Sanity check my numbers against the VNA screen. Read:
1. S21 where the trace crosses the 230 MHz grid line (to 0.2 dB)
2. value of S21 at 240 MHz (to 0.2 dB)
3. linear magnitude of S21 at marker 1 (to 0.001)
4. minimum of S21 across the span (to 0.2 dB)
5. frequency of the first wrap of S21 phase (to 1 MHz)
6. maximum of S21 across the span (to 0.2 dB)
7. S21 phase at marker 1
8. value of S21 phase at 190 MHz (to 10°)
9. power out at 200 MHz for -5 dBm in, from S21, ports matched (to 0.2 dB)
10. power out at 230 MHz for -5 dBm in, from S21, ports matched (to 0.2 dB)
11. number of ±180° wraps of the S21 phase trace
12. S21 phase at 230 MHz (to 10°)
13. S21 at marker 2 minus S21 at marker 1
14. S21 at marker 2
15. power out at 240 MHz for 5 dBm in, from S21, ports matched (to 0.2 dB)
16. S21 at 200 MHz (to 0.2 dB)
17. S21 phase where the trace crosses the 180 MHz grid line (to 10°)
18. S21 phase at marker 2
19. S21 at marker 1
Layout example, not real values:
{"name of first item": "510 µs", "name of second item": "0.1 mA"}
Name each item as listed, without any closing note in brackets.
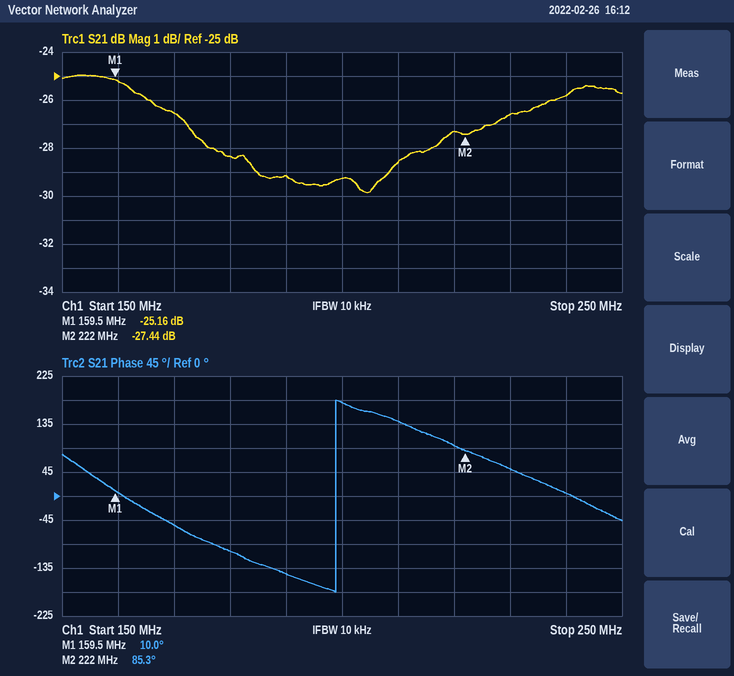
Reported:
{"S21 where the trace crosses the 230 MHz grid line": "-26.6 dB", "value of S21 at 240 MHz": "-25.8 dB", "linear magnitude of S21 at marker 1": "0.055", "minimum of S21 across the span": "-29.8 dB", "frequency of the first wrap of S21 phase": "199 MHz", "maximum of S21 across the span": "-25.0 dB", "S21 phase at marker 1": "10.0°", "value of S21 phase at 190 MHz": "-150°", "power out at 200 MHz for -5 dBm in, from S21, ports matched": "-34.2 dBm", "power out at 230 MHz for -5 dBm in, from S21, ports matched": "-31.6 dBm", "number of ±180° wraps of the S21 phase trace": "1", "S21 phase at 230 MHz": "50°", "S21 at marker 2 minus S21 at marker 1": "-2.28 dB", "S21 at marker 2": "-27.44 dB", "power out at 240 MHz for 5 dBm in, from S21, ports matched": "-20.8 dBm", "S21 at 200 MHz": "-29.2 dB", "S21 phase where the trace crosses the 180 MHz grid line": "-100°", "S21 phase at marker 2": "85.3°", "S21 at marker 1": "-25.16 dB"}
